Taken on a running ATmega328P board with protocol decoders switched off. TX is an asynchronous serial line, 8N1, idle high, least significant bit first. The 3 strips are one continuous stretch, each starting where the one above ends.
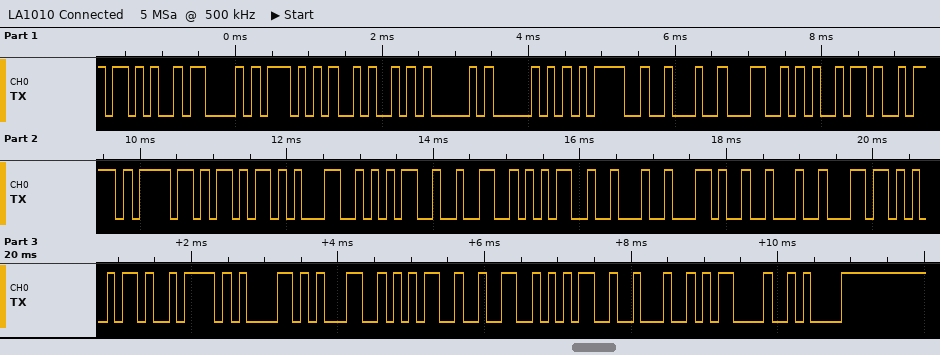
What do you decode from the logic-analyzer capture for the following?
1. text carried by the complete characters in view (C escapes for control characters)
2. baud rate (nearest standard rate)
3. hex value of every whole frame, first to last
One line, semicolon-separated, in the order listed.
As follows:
"+CWJAP=\"Lizok1525\",\"liza1525\"\r\n"; 9600 baud; 2B 43 57 4A 41 50 3D 22 4C 69 7A 6F 6B 31 35 32 35 22 2C 22 6C 69 7A 61 31 35 32 35 22 0D 0A
